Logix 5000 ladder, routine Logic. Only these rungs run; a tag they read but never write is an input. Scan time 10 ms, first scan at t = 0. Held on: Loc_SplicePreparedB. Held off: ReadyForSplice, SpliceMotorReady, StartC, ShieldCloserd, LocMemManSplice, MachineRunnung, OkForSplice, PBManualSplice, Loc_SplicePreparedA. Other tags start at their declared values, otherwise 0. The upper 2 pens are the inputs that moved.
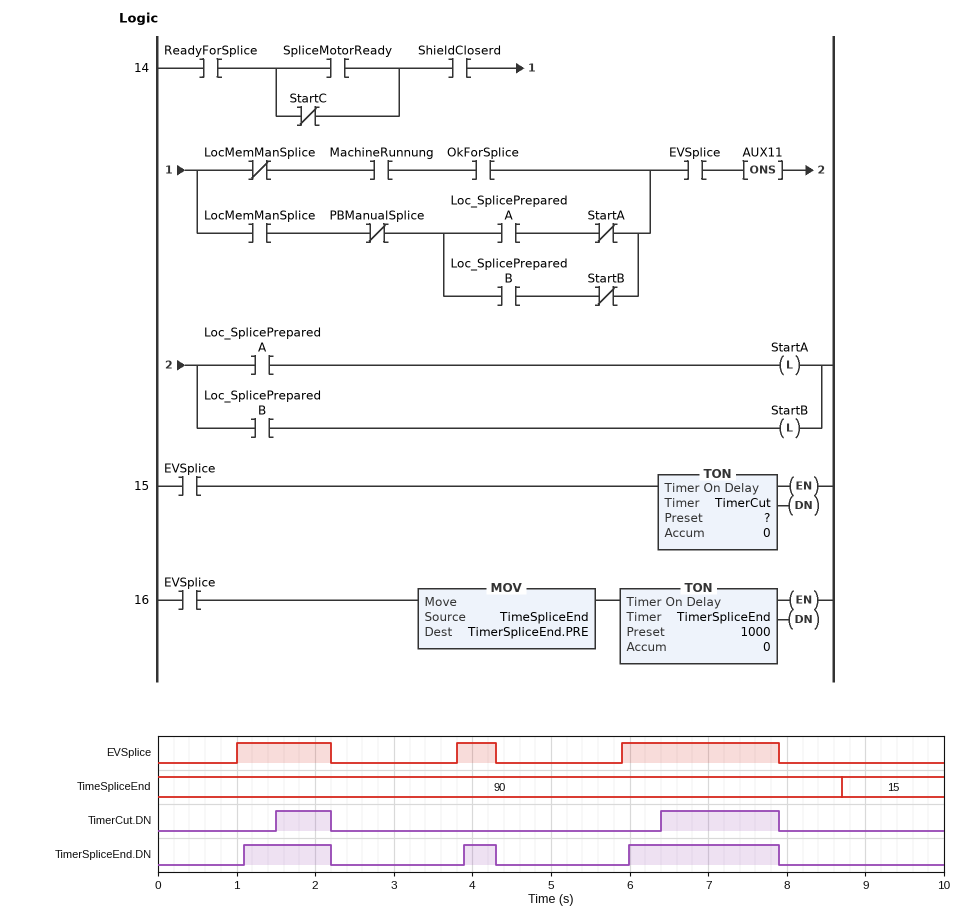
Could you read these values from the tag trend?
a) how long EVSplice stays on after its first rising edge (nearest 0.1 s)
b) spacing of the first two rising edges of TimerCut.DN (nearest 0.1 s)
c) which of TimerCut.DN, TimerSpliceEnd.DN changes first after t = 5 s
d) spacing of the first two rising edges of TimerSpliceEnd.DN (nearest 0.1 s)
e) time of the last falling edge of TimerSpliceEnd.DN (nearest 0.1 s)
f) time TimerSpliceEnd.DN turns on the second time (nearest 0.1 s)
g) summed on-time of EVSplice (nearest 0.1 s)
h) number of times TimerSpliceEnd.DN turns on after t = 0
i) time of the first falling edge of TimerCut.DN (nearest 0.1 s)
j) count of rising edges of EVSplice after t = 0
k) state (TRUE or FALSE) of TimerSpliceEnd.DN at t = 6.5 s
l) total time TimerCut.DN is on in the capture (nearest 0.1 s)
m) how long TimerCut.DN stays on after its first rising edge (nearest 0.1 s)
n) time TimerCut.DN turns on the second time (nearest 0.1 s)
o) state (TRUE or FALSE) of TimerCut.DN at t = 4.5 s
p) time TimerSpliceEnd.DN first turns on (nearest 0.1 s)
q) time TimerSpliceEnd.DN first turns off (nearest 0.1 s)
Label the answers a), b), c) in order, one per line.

a) 1.2 s
b) 4.9 s
c) TimerSpliceEnd.DN
d) 2.8 s
e) 7.9 s
f) 3.9 s
g) 3.7 s
h) 3
i) 2.2 s
j) 3
k) TRUE
l) 2.2 s
m) 0.7 s
n) 6.4 s
o) FALSE
p) 1.1 s
q) 2.2 s
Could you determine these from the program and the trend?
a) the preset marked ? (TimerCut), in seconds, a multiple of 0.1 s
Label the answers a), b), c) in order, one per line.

a) 0.5 s
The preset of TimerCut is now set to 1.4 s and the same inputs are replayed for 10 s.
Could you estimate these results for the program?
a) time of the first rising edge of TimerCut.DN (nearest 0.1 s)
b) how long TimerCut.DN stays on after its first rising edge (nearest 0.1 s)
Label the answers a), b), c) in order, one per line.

a) 7.3 s
b) 0.6 s
